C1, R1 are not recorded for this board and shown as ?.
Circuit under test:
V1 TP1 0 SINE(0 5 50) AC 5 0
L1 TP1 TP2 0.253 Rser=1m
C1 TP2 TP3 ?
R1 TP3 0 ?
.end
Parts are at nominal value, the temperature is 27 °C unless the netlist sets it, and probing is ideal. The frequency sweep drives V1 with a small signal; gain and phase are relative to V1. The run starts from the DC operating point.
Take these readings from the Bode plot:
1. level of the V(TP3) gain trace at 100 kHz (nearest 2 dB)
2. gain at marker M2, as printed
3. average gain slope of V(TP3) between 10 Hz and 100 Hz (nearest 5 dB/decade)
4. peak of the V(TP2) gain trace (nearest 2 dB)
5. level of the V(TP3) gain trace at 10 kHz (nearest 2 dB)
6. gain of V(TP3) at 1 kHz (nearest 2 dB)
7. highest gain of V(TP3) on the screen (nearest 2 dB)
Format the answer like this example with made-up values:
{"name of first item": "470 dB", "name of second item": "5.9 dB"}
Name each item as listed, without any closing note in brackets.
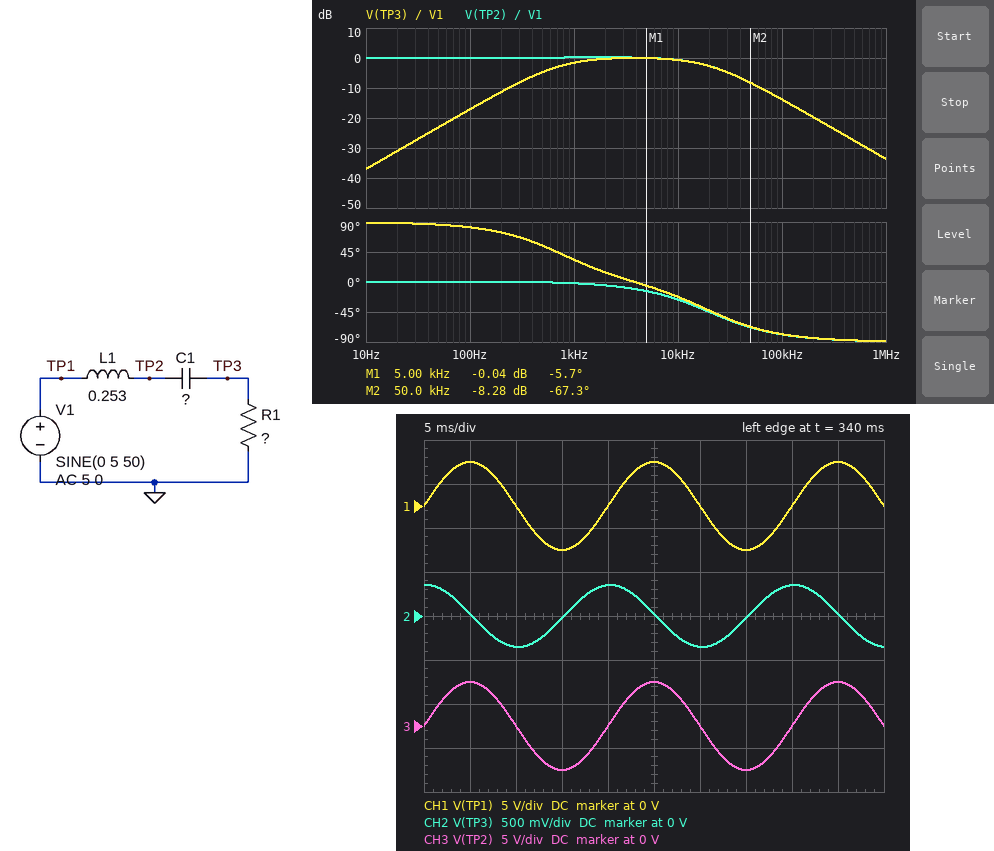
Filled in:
{"level of the V(TP3) gain trace at 100 kHz": "-14 dB", "gain at marker M2, as printed": "-8.28 dB", "average gain slope of V(TP3) between 10 Hz and 100 Hz": "20 dB/decade", "peak of the V(TP2) gain trace": "0 dB", "level of the V(TP3) gain trace at 10 kHz": "0 dB", "gain of V(TP3) at 1 kHz": "-2 dB", "highest gain of V(TP3) on the screen": "0 dB"}
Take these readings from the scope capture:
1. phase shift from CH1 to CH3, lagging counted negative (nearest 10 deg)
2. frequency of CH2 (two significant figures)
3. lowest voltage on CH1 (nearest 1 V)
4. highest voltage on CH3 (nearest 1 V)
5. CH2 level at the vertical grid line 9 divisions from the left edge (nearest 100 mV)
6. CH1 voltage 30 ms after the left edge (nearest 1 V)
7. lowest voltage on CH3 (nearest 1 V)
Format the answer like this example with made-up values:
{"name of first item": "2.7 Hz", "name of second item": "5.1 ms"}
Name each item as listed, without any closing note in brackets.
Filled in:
{"phase shift from CH1 to CH3, lagging counted negative": "0 deg", "frequency of CH2": "50 Hz", "lowest voltage on CH1": "-5 V", "highest voltage on CH3": "5 V", "CH2 level at the vertical grid line 9 divisions from the left edge": "0 V", "CH1 voltage 30 ms after the left edge": "0 V", "lowest voltage on CH3": "-5 V"}
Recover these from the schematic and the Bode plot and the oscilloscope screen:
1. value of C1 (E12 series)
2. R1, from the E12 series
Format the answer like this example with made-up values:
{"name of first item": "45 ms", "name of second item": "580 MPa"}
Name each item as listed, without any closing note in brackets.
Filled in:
{"value of C1": "6.8 nF", "R1, from the E12 series": "33 kΩ"}
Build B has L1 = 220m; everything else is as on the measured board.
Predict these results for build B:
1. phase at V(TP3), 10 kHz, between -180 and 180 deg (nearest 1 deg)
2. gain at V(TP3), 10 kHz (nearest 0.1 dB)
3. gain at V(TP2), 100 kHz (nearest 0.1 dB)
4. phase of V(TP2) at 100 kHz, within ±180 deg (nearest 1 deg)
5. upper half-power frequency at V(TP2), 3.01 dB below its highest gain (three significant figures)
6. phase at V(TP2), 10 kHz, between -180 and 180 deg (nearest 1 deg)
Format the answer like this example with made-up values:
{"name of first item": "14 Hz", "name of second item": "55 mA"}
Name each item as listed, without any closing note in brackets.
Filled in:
{"phase at V(TP3), 10 kHz, between -180 and 180 deg": "-19 deg", "gain at V(TP3), 10 kHz": "-0.5 dB", "gain at V(TP2), 100 kHz": "-12.7 dB", "phase of V(TP2) at 100 kHz, within ±180 deg": "-77 deg", "upper half-power frequency at V(TP2), 3.01 dB below its highest gain": "23.5 kHz", "phase at V(TP2), 10 kHz, between -180 and 180 deg": "-23 deg"}
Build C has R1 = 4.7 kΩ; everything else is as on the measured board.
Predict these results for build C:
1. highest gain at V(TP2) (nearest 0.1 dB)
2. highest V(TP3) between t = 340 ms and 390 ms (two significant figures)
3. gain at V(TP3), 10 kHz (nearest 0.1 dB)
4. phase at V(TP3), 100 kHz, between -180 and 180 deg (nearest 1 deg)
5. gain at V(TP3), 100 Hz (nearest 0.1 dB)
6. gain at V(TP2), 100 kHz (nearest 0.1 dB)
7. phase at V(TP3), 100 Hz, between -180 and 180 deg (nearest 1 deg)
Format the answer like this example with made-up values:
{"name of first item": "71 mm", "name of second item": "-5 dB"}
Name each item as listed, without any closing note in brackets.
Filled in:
{"highest gain at V(TP2)": "4.6 dB", "highest V(TP3) between t = 340 ms and 390 ms": "50 mV", "gain at V(TP3), 10 kHz": "-9.7 dB", "phase at V(TP3), 100 kHz, between -180 and 180 deg": "-88 deg", "gain at V(TP3), 100 Hz": "-33.9 dB", "gain at V(TP2), 100 kHz": "-30.6 dB", "phase at V(TP3), 100 Hz, between -180 and 180 deg": "89 deg"}
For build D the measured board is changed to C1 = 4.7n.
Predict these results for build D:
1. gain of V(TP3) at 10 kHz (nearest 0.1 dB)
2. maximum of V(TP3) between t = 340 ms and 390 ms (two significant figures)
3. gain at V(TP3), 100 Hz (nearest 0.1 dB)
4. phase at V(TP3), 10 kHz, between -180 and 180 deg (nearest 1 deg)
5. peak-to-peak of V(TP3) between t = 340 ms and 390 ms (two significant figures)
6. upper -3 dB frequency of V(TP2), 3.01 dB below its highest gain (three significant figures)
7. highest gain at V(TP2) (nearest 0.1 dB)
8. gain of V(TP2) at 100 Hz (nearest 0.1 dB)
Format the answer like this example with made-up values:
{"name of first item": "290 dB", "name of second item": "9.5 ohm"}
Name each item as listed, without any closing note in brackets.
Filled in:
{"gain of V(TP3) at 10 kHz": "-0.6 dB", "maximum of V(TP3) between t = 340 ms and 390 ms": "240 mV", "gain at V(TP3), 100 Hz": "-20.3 dB", "phase at V(TP3), 10 kHz, between -180 and 180 deg": "-21 deg", "peak-to-peak of V(TP3) between t = 340 ms and 390 ms": "490 mV", "upper -3 dB frequency of V(TP2), 3.01 dB below its highest gain": "20.3 kHz", "highest gain at V(TP2)": "0.3 dB", "gain of V(TP2) at 100 Hz": "0 dB"}
